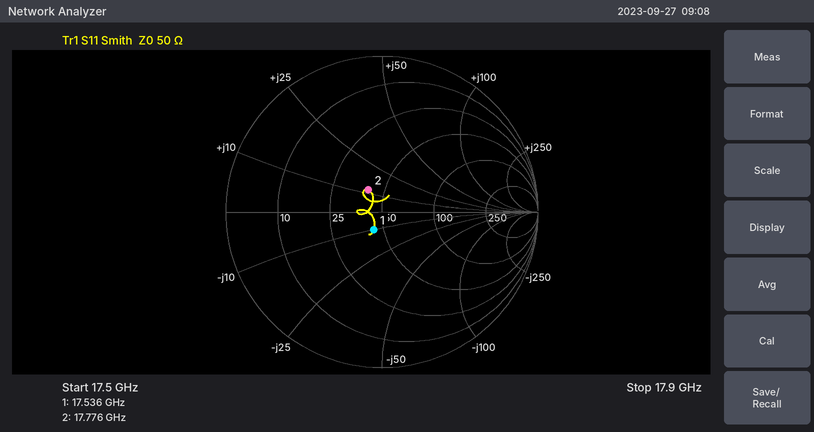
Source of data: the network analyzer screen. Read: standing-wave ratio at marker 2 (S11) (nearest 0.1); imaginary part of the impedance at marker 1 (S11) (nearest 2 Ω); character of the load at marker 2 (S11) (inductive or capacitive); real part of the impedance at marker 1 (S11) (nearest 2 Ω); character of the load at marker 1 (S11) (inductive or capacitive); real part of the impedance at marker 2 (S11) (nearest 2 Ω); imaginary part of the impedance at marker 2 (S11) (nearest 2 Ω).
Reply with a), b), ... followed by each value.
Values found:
a) 1.4
b) -10 Ω
c) inductive
d) 44 Ω
e) capacitive
f) 40 Ω
g) +12 Ω
